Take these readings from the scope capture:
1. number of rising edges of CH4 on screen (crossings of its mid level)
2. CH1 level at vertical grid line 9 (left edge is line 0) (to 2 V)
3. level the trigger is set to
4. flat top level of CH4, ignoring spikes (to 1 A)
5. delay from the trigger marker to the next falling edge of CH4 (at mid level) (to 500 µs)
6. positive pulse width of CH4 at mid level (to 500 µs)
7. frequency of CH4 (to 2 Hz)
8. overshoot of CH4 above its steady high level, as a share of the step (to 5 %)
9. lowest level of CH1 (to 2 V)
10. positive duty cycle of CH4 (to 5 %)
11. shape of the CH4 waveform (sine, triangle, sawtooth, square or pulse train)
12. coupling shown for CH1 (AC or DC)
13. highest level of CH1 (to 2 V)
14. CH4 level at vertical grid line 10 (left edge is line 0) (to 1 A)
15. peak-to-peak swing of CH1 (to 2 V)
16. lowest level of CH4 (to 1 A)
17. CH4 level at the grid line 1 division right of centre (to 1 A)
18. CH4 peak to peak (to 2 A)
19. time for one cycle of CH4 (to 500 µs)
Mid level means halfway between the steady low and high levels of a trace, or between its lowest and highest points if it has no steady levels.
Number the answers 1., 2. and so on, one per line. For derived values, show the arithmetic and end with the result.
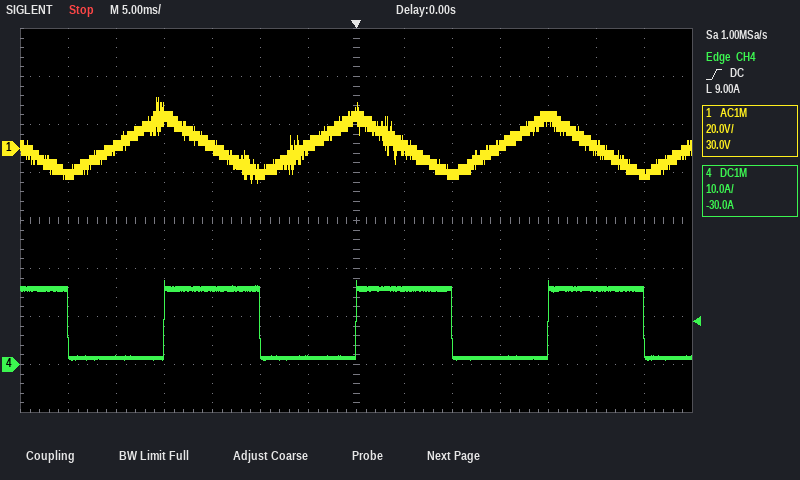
1. 3
2. -10 V
3. 9.00 A
4. 16 A
5. 10.0 ms
6. 10.0 ms
7. 1 / 20.0 ms ≈ 50 Hz
8. 10 %
9. -14 V
10. 10.0 ms / 20.0 ms ≈ 50 %
11. square
12. AC
13. 22 V
14. 1 A
15. 22 V − (-14 V) = 36 V
16. 1 A
17. 16 A
18. 16 A
19. 20.0 ms
